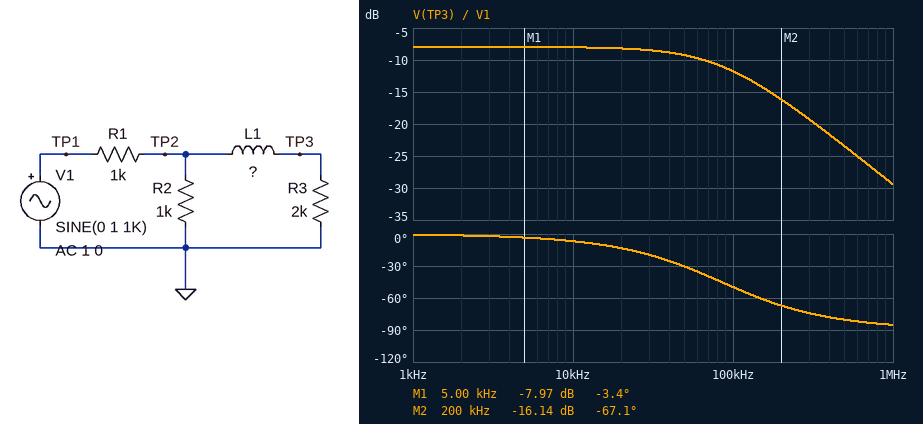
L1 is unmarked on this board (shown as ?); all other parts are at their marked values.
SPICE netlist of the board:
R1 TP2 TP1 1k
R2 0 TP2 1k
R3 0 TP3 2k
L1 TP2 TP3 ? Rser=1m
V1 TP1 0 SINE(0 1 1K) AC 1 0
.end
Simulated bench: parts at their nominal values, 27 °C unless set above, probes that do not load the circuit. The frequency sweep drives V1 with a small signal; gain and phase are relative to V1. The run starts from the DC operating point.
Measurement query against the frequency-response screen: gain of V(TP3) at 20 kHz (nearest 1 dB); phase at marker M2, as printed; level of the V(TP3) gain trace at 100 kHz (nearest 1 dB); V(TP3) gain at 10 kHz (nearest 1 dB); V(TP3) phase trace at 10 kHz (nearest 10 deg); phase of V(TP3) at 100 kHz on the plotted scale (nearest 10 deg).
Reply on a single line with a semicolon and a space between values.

-8 dB; -67.1 deg; -12 dB; -8 dB; -10 deg; -50 deg
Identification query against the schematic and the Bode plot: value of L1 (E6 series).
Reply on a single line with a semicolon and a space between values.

4.7 mH
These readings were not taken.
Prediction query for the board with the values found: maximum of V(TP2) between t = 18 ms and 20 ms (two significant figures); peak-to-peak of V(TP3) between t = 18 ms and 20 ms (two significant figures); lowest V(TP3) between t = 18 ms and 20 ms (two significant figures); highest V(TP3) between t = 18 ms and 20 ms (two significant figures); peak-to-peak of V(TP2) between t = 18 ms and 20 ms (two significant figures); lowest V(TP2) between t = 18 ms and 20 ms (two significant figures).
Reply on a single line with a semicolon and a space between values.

400 mV; 800 mV; -400 mV; 400 mV; 800 mV; -400 mV
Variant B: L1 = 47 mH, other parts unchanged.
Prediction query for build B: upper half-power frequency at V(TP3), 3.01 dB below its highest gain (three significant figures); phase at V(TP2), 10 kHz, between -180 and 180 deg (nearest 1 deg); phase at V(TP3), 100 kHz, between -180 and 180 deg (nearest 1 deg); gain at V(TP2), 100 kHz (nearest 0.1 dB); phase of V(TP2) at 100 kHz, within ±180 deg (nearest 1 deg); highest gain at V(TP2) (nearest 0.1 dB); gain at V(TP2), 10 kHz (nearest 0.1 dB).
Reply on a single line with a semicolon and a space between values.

8.47 kHz; 6 deg; -85 deg; -6.0 dB; 1 deg; -6.0 dB; -6.7 dB
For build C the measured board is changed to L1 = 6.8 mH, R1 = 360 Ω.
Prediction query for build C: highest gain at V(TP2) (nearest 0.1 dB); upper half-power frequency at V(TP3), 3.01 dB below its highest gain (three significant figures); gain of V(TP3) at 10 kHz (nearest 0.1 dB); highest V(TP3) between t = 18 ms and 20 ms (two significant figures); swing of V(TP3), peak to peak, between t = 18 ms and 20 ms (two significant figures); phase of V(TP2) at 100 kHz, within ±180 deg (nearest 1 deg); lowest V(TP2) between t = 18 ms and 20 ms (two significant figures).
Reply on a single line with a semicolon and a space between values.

-2.7 dB; 53.0 kHz; -3.9 dB; 650 mV; 1.3 V; 3 deg; -650 mV
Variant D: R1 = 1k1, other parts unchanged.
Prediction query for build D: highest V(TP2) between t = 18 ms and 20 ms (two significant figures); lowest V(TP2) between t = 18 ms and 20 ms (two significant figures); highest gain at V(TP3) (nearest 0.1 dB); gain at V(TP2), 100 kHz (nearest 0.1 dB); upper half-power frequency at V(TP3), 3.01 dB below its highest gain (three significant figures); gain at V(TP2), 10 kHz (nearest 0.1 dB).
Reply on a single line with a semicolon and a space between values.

380 mV; -380 mV; -8.5 dB; -7.2 dB; 85.5 kHz; -8.4 dB
